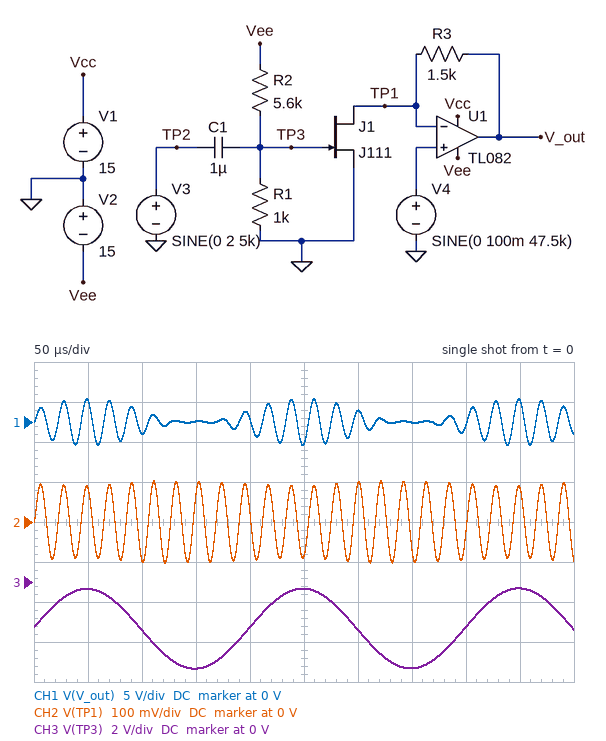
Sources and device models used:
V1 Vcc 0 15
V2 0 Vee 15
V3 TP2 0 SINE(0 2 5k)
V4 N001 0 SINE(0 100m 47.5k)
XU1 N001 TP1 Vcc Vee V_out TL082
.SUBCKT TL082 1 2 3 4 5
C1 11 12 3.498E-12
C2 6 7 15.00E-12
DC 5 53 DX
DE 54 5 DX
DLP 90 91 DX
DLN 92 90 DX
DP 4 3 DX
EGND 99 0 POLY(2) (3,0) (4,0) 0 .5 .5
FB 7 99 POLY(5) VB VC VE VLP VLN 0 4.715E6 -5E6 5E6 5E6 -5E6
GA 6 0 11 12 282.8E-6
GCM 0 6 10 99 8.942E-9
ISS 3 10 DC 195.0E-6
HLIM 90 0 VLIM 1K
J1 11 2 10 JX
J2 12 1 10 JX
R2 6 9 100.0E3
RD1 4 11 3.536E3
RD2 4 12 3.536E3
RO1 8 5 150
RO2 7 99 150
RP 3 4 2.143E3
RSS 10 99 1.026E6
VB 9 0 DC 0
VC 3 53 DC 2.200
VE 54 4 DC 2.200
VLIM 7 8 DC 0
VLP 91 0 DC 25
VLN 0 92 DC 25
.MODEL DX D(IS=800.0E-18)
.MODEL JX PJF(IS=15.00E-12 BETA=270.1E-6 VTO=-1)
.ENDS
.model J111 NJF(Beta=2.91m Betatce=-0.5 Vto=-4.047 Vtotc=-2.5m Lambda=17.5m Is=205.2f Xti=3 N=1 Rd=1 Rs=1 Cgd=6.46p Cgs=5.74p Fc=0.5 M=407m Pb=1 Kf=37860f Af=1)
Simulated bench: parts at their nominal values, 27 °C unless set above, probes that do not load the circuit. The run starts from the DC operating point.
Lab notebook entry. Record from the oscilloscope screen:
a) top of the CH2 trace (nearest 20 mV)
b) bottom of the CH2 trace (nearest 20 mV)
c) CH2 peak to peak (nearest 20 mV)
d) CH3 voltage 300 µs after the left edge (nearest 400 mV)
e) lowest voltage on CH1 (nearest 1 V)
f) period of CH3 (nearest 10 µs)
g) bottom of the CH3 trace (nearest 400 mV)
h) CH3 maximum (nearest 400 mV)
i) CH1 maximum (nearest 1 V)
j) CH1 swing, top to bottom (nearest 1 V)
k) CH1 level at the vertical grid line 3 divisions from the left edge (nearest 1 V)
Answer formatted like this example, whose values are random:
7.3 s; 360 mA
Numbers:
100 mV; -100 mV; 200 mV; -2.4 V; -3 V; 200 µs; -4.4 V; -400 mV; 3 V; 6 V; 0 V
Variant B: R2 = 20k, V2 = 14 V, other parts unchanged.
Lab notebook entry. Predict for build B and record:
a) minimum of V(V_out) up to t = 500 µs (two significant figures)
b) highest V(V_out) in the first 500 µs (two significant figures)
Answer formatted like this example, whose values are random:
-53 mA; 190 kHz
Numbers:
-12 V; 3.2 V
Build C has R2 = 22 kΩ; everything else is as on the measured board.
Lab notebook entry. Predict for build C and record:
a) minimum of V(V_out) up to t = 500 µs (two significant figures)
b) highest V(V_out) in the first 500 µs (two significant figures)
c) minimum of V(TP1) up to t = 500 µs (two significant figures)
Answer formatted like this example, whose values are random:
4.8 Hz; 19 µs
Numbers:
-13 V; 3.2 V; -100 mV
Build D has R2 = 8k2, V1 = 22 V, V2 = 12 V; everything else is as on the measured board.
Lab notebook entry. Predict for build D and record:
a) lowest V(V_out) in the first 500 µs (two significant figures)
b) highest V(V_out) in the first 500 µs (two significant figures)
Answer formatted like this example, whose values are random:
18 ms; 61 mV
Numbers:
-8.9 V; 3.3 V
